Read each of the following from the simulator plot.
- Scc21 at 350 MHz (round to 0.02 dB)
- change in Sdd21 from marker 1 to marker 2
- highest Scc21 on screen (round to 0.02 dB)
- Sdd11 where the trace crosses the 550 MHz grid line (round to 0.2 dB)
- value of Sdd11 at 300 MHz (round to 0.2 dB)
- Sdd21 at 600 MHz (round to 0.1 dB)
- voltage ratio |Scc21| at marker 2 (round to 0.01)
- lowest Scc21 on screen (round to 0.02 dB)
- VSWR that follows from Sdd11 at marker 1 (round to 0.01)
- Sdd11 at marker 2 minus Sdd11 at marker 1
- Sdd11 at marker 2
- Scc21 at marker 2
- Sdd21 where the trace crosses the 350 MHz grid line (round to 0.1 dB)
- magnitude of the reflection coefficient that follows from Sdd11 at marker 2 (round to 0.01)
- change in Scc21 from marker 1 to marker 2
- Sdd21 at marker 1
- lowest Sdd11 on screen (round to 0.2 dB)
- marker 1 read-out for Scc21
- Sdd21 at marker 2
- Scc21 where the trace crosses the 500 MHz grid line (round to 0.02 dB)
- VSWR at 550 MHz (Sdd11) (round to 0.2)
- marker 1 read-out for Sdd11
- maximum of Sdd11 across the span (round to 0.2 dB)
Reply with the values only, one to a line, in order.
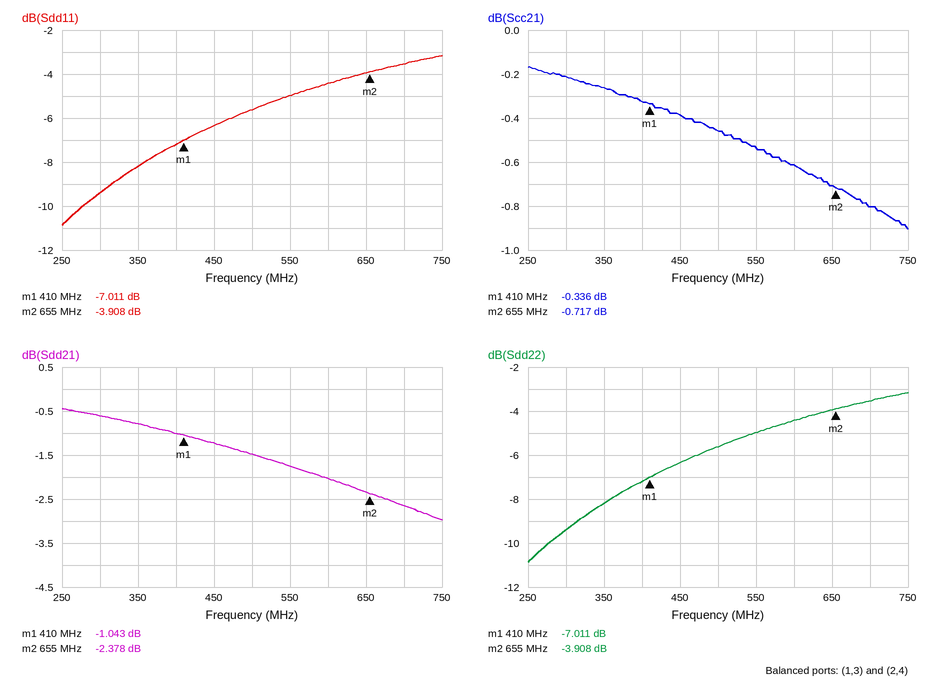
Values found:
-0.26 dB
-1.335 dB
-0.16 dB
-5.0 dB
-9.4 dB
-2.0 dB
0.92
-0.90 dB
2.61
3.103 dB
-3.908 dB
-0.717 dB
-0.8 dB
0.64
-0.381 dB
-1.043 dB
-10.8 dB
-0.336 dB
-2.378 dB
-0.46 dB
3.6
-7.011 dB
-3.2 dB
